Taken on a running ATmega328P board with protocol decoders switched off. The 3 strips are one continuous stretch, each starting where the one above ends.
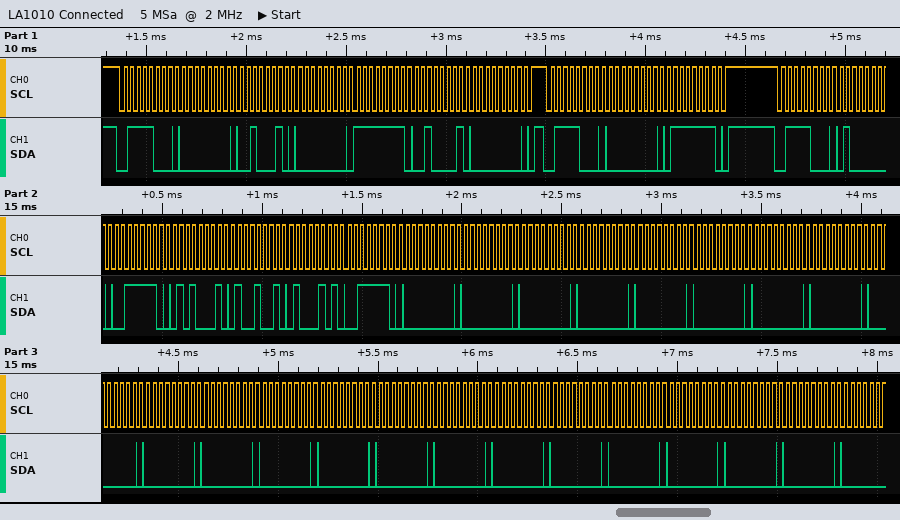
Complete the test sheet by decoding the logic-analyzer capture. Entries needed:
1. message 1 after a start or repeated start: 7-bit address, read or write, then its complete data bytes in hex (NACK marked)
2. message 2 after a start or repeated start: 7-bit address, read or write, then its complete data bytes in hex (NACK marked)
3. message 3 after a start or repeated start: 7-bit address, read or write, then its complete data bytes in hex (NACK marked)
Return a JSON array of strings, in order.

["0x3C write: 00 22 00 FF 21 00", "0x3C write: 00 7F", "0x3C write: 40 3E 51 49 45 3E 00 00 00 00 00 00 00 00 00 00 00 00 00 00 00 00 00 00 00 00 00"]
